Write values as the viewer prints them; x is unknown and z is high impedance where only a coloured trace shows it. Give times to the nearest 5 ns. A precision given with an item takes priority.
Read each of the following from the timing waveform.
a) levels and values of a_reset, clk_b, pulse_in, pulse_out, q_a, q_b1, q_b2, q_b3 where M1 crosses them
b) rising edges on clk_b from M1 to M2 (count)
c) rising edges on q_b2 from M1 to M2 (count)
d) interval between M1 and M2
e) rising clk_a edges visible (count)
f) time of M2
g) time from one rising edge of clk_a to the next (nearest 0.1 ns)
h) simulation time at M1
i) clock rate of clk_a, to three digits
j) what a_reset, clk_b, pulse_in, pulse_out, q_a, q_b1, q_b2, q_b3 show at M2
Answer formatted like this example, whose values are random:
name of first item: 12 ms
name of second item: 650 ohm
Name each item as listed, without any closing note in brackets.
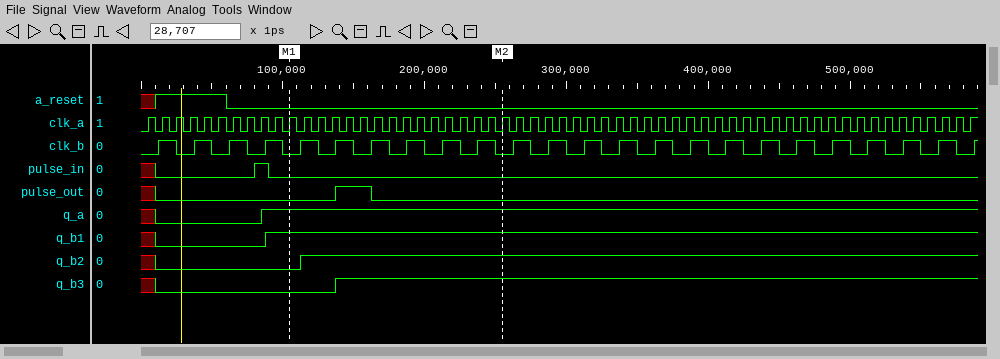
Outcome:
levels and values of a_reset, clk_b, pulse_in, pulse_out, q_a, q_b1, q_b2, q_b3 where M1 crosses them: a_reset=0, clk_b=0, pulse_in=0, pulse_out=0, q_a=1, q_b1=1, q_b2=0, q_b3=0
rising edges on clk_b from M1 to M2: 6
rising edges on q_b2 from M1 to M2: 1
interval between M1 and M2: 150 ns
rising clk_a edges visible: 59
time of M2: 255 ns
time from one rising edge of clk_a to the next: 10 ns
simulation time at M1: 105 ns
clock rate of clk_a, to three digits: 100 MHz
what a_reset, clk_b, pulse_in, pulse_out, q_a, q_b1, q_b2, q_b3 show at M2: a_reset=0, clk_b=0, pulse_in=0, pulse_out=0, q_a=1, q_b1=1, q_b2=1, q_b3=1
